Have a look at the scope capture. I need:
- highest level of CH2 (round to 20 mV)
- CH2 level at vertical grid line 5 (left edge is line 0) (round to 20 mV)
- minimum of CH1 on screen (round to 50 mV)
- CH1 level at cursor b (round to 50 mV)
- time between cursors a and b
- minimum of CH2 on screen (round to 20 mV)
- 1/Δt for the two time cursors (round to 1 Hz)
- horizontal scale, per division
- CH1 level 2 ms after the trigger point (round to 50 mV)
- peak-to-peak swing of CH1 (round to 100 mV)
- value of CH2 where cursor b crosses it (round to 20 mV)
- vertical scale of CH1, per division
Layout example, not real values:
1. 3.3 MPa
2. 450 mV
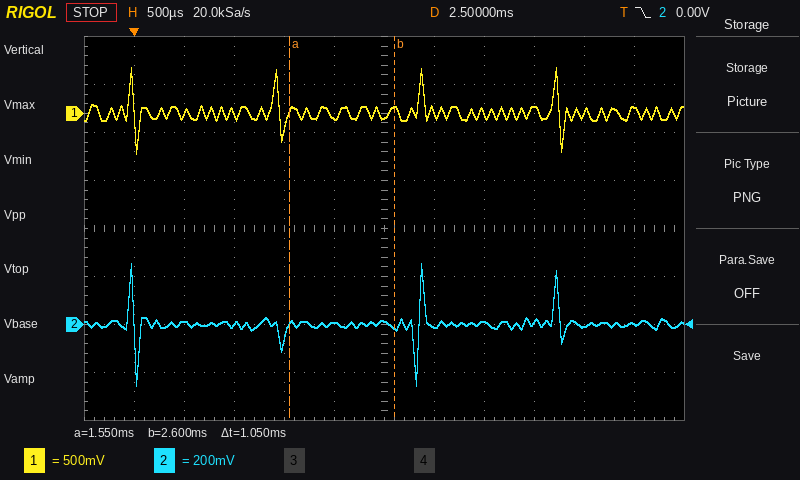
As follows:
1. 260 mV
2. 0 mV
3. -400 mV
4. 50 mV
5. 1.05 ms
6. -260 mV
7. 952 Hz
8. 500 µs
9. -50 mV
10. 900 mV
11. -20 mV
12. 500 mV
